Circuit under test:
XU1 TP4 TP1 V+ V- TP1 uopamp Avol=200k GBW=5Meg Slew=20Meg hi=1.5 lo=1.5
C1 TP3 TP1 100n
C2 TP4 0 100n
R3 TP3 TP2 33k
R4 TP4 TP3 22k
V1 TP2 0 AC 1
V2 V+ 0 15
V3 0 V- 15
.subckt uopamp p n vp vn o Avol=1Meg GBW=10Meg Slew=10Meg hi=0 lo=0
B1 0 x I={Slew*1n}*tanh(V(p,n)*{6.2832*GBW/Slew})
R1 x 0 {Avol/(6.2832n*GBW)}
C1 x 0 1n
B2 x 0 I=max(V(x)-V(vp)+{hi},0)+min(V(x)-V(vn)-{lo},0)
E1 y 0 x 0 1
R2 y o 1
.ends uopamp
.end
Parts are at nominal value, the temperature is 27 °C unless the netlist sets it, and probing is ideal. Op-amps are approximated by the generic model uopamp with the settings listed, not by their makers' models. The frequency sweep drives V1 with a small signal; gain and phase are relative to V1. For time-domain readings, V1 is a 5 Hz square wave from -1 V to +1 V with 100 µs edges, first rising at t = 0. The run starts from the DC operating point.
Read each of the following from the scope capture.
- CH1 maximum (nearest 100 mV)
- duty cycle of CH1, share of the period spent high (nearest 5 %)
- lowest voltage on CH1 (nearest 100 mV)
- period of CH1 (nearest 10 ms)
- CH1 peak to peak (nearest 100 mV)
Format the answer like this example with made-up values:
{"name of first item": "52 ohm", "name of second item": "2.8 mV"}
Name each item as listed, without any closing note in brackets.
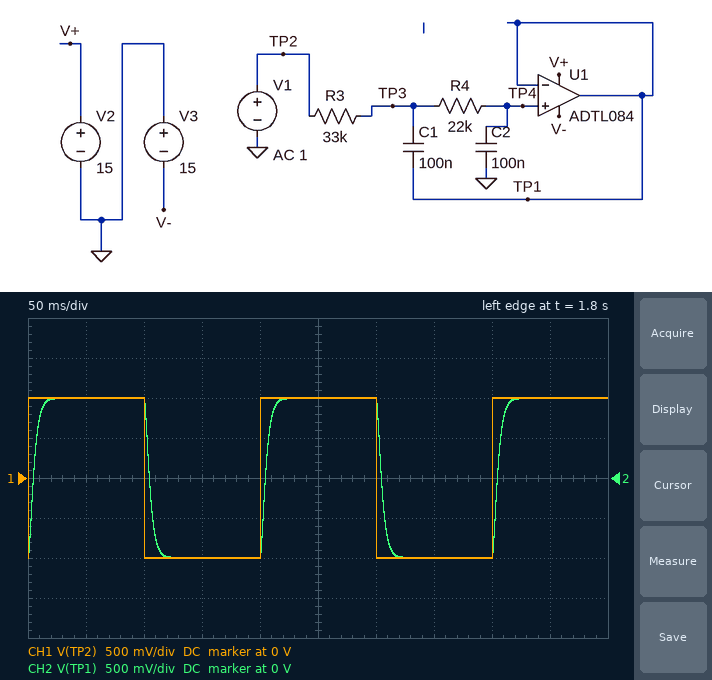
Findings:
{"CH1 maximum": "1.0 V", "duty cycle of CH1, share of the period spent high": "50 %", "lowest voltage on CH1": "-1.0 V", "period of CH1": "200 ms", "CH1 peak to peak": "2.0 V"}
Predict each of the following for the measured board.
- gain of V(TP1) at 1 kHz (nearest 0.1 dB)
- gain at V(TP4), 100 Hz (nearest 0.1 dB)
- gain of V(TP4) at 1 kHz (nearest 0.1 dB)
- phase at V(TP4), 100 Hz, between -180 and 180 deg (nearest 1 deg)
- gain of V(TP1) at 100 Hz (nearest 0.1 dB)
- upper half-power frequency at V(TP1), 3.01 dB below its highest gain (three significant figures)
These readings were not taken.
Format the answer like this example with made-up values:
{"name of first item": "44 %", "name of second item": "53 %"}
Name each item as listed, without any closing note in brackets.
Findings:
{"gain of V(TP1) at 1 kHz": "-49.2 dB", "gain at V(TP4), 100 Hz": "-11.9 dB", "gain of V(TP4) at 1 kHz": "-49.2 dB", "phase at V(TP4), 100 Hz, between -180 and 180 deg": "-118 deg", "gain of V(TP1) at 100 Hz": "-11.9 dB", "upper half-power frequency at V(TP1), 3.01 dB below its highest gain": "36.9 Hz"}
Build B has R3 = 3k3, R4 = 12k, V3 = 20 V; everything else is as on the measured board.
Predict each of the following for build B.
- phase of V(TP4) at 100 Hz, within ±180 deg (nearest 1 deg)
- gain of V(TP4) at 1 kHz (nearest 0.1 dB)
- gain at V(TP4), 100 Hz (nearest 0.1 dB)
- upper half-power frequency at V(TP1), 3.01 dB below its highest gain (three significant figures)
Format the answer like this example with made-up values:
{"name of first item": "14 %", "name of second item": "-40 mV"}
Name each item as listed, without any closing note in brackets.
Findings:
{"phase of V(TP4) at 100 Hz, within ±180 deg": "-49 deg", "gain of V(TP4) at 1 kHz": "-24.9 dB", "gain at V(TP4), 100 Hz": "-2.1 dB", "upper half-power frequency at V(TP1), 3.01 dB below its highest gain": "124 Hz"}
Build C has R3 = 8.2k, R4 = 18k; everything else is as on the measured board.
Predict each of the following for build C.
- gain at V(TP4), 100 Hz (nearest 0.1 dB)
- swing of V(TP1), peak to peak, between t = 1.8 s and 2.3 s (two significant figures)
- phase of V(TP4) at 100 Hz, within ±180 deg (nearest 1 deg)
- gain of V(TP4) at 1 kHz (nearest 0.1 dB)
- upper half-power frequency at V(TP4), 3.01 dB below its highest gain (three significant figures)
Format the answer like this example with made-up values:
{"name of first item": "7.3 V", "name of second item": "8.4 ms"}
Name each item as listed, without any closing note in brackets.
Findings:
{"gain at V(TP4), 100 Hz": "-4.6 dB", "swing of V(TP1), peak to peak, between t = 1.8 s and 2.3 s": "2.0 V", "phase of V(TP4) at 100 Hz, within ±180 deg": "-76 deg", "gain of V(TP4) at 1 kHz": "-35.5 dB", "upper half-power frequency at V(TP4), 3.01 dB below its highest gain": "75.8 Hz"}
